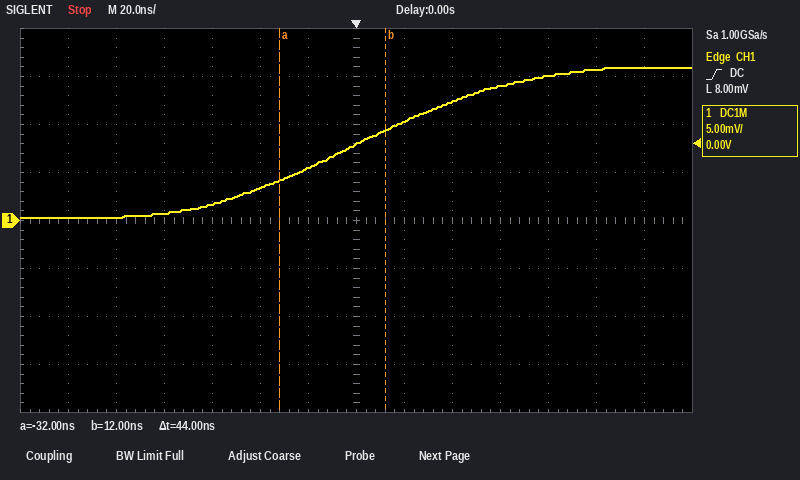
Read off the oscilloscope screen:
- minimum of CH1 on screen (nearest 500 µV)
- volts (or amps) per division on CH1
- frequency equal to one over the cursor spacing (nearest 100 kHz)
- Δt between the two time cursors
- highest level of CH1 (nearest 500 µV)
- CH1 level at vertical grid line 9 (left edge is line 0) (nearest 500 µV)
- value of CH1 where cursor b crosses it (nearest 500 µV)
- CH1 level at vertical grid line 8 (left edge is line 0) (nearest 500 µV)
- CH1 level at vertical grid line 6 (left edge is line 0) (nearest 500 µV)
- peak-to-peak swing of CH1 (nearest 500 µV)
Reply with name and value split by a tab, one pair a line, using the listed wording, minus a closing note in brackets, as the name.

minimum of CH1 on screen	500 µV
volts (or amps) per division on CH1	5 mV
frequency equal to one over the cursor spacing	22.7 MHz
Δt between the two time cursors	44 ns
highest level of CH1	16.0 mV
CH1 level at vertical grid line 9 (left edge is line 0)	12.5 mV
value of CH1 where cursor b crosses it	9.5 mV
CH1 level at vertical grid line 8 (left edge is line 0)	10.5 mV
CH1 level at vertical grid line 6 (left edge is line 0)	5.5 mV
peak-to-peak swing of CH1	15.5 mV
